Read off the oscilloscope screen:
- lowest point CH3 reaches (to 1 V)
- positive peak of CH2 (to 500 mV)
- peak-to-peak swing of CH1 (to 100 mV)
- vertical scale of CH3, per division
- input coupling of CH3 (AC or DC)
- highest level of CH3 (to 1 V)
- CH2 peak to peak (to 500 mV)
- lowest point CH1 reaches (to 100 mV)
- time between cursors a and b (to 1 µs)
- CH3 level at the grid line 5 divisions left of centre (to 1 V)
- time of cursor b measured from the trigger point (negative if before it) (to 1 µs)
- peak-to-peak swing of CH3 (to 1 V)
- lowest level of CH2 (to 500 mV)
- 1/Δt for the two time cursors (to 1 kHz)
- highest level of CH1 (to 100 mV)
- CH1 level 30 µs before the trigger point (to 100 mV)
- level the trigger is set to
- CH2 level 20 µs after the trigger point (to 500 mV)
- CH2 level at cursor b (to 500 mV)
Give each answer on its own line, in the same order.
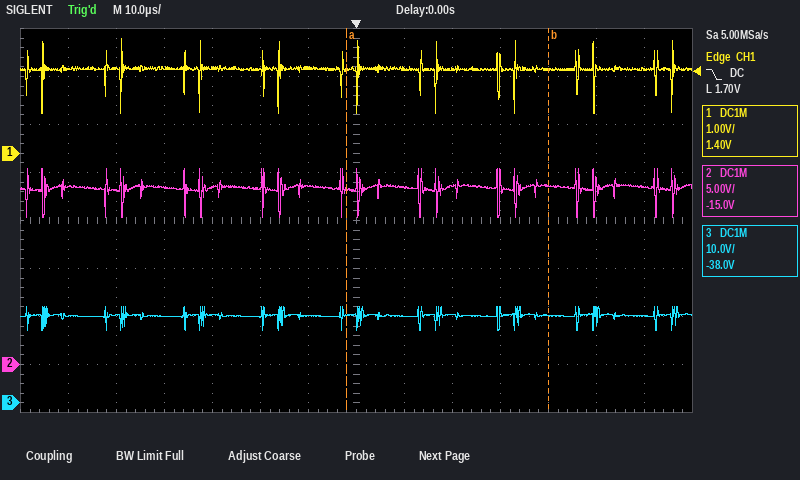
15 V
20.5 V
1.6 V
10 V
DC
20 V
5.0 V
800 mV
42 µs
18 V
+40 µs
5 V
15.5 V
24 kHz
2.4 V
1.8 V
1.70 V
18.5 V
18.5 V
